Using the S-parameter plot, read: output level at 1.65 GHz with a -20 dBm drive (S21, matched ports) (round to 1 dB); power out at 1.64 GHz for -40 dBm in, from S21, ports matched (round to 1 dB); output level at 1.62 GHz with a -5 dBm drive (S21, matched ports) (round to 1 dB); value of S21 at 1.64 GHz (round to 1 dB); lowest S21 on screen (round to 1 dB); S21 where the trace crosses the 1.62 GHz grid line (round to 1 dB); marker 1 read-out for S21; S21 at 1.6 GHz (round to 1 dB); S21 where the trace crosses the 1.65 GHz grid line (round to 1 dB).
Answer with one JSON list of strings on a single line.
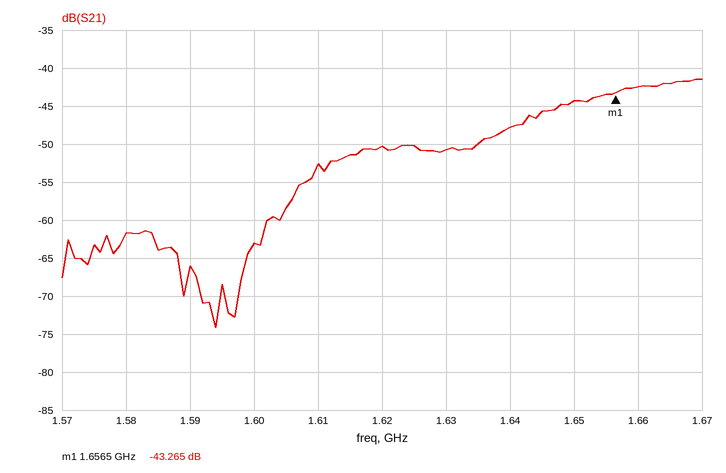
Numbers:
["-64 dBm", "-88 dBm", "-55 dBm", "-48 dB", "-74 dB", "-50 dB", "-43.265 dB", "-63 dB", "-44 dB"]
